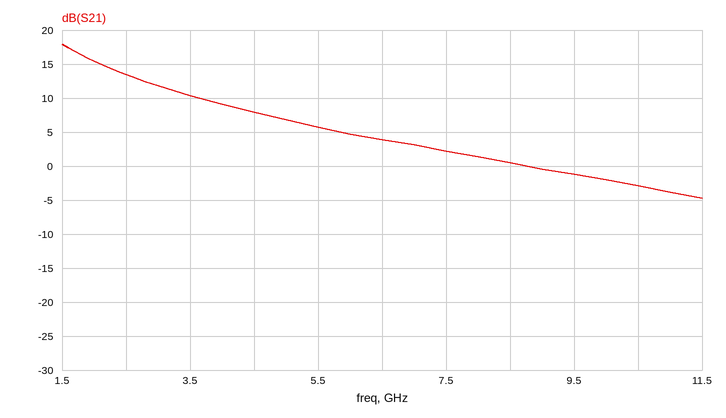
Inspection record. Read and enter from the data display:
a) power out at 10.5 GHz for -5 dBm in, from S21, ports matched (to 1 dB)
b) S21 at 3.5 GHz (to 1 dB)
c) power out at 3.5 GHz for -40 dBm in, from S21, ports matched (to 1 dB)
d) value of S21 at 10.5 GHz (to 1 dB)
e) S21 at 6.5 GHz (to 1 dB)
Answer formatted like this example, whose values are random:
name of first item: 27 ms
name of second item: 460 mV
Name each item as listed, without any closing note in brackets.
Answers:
power out at 10.5 GHz for -5 dBm in, from S21, ports matched: -8 dBm
S21 at 3.5 GHz: 10 dB
power out at 3.5 GHz for -40 dBm in, from S21, ports matched: -30 dBm
value of S21 at 10.5 GHz: -3 dB
S21 at 6.5 GHz: 4 dB
